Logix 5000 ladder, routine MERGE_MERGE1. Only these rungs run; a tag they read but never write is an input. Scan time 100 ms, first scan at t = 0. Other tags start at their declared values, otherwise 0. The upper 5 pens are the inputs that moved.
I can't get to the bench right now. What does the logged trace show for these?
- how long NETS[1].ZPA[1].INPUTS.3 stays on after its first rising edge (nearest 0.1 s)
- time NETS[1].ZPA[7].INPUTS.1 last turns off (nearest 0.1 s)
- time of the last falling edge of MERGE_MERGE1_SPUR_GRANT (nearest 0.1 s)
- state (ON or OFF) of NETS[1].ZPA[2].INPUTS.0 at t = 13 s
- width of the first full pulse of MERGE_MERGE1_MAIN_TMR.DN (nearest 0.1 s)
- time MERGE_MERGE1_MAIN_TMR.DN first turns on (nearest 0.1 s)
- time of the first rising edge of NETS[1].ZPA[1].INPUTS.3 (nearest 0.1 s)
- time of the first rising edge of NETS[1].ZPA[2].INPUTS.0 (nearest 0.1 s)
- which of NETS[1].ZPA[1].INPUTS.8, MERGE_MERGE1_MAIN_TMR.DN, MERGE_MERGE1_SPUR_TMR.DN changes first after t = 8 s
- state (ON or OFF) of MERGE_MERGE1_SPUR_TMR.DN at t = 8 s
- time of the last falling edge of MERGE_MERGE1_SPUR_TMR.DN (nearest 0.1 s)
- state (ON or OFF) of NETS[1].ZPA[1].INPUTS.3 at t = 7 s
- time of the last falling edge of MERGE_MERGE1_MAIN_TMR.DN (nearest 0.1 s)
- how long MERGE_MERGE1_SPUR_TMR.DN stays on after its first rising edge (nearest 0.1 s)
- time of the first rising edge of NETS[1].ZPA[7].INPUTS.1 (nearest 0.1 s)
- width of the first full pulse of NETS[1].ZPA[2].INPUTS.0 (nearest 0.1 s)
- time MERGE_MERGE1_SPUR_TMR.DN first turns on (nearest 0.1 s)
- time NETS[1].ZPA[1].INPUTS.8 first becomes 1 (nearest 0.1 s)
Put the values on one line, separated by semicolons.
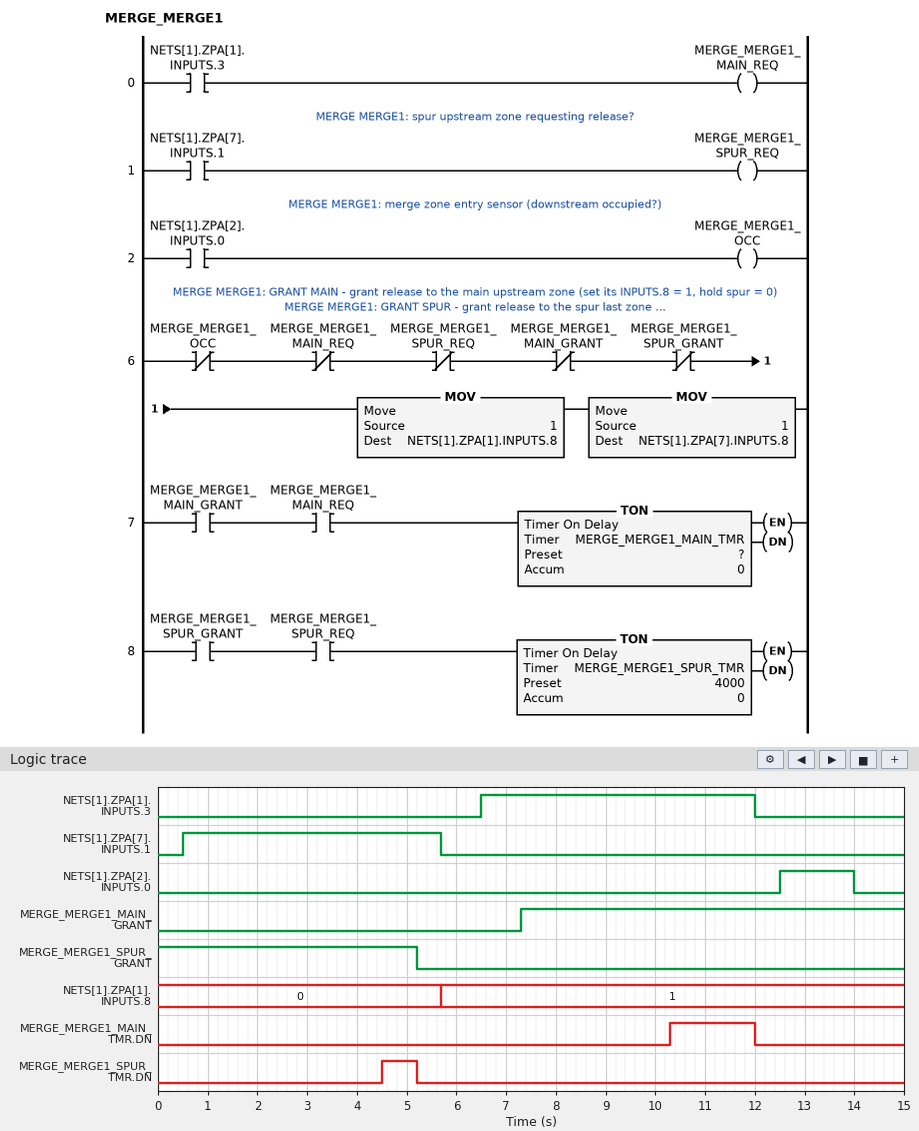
5.5 s; 5.7 s; 5.2 s; ON; 1.7 s; 10.3 s; 6.5 s; 12.5 s; MERGE_MERGE1_MAIN_TMR.DN; OFF; 5.2 s; ON; 12.0 s; 0.7 s; 0.5 s; 1.5 s; 4.5 s; 5.7 s
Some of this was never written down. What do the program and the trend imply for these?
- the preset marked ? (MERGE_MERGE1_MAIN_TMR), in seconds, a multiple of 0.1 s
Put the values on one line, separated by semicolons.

3.0 s
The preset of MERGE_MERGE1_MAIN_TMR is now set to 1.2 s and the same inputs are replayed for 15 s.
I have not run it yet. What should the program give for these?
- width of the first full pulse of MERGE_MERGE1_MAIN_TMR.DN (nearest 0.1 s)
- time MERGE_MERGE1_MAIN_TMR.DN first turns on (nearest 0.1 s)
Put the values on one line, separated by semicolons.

3.5 s; 8.5 s
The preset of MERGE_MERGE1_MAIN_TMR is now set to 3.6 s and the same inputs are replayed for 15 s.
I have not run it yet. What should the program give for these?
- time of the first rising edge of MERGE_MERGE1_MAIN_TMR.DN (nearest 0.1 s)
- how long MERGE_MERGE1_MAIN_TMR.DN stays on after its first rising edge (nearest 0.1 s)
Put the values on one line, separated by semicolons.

10.9 s; 1.1 s
